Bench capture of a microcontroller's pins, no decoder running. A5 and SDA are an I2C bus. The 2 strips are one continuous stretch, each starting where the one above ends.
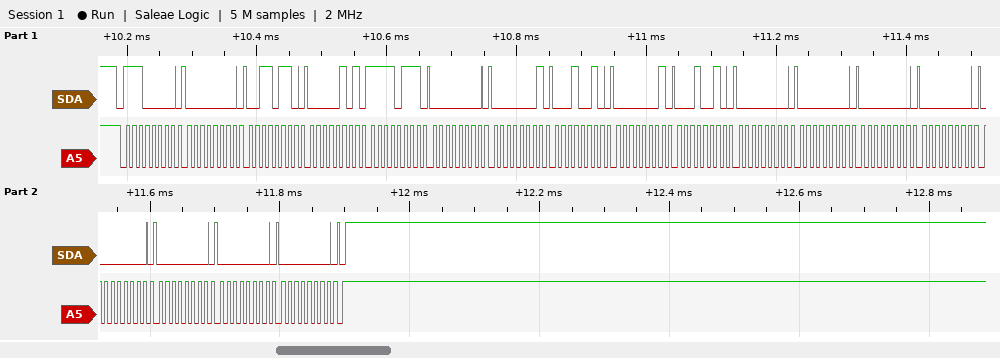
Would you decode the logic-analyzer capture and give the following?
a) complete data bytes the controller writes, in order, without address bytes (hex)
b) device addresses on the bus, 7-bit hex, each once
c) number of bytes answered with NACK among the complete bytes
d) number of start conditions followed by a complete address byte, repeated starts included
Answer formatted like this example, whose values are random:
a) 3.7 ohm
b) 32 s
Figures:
a) 00 36 05 F7 00 01 12 01 12 00 00 00 00 00 00 00 00
b) 0x70
c) 0
d) 1
